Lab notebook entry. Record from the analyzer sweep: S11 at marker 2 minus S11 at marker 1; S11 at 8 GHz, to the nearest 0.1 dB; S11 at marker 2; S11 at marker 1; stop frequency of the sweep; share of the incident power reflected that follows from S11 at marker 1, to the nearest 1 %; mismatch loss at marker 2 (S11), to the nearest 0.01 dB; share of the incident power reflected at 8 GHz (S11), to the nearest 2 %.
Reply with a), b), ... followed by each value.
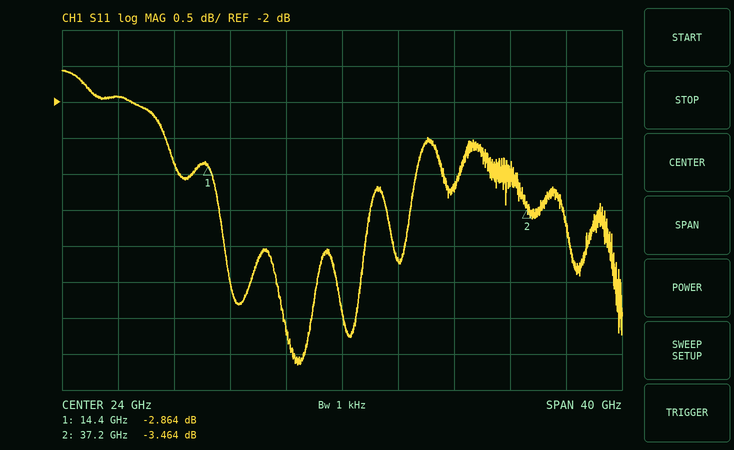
a) -0.600 dB
b) -1.9 dB
c) -3.464 dB
d) -2.864 dB
e) 44 GHz
f) 52 %
g) 2.60 dB
h) 64 %
